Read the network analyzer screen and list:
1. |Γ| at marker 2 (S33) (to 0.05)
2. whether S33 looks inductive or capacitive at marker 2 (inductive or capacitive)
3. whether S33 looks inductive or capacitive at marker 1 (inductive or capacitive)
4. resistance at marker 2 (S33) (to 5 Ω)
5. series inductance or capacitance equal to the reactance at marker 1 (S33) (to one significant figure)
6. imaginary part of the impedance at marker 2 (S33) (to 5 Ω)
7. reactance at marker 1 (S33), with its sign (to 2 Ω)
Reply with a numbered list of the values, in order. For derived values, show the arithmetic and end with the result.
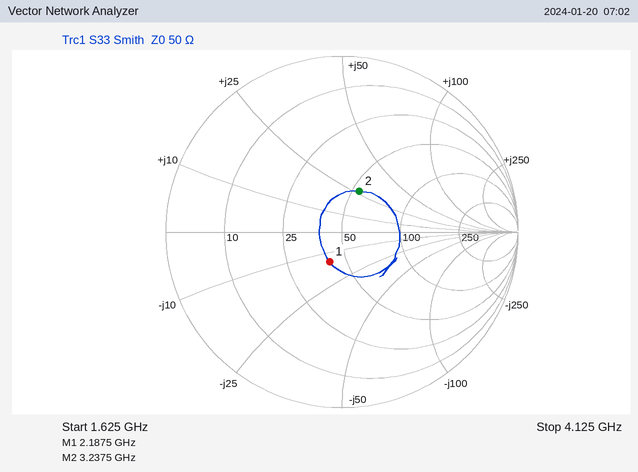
1. 0.25
2. inductive
3. capacitive
4. 55 Ω
5. C = 1/(2π × 2.1875 GHz × 14 Ω) ≈ 5 pF
6. +25 Ω
7. -14 Ω
